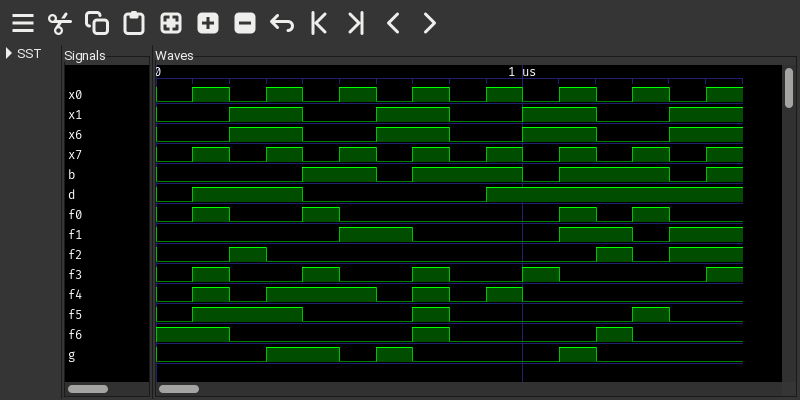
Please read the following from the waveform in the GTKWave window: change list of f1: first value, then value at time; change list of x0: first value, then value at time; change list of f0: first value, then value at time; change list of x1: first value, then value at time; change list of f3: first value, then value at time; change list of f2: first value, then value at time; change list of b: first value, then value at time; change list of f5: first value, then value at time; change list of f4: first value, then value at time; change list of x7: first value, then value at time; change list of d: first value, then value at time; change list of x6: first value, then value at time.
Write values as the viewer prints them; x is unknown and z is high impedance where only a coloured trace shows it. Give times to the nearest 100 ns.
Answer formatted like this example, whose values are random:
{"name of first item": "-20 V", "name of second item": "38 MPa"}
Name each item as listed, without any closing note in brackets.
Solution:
{"change list of f1: first value, then value at time": "0, 1 at 500 ns, 0 at 700 ns, 1 at 1100 ns, 0 at 1300 ns, 1 at 1400 ns", "change list of x0: first value, then value at time": "0, 1 at 100 ns, 0 at 200 ns, 1 at 300 ns, 0 at 400 ns, 1 at 500 ns, 0 at 600 ns, 1 at 700 ns, 0 at 800 ns, 1 at 900 ns, 0 at 1000 ns, 1 at 1100 ns, 0 at 1200 ns, 1 at 1300 ns, 0 at 1400 ns, 1 at 1500 ns", "change list of f0: first value, then value at time": "0, 1 at 100 ns, 0 at 200 ns, 1 at 400 ns, 0 at 500 ns, 1 at 1100 ns, 0 at 1200 ns, 1 at 1300 ns, 0 at 1400 ns", "change list of x1: first value, then value at time": "0, 1 at 200 ns, 0 at 400 ns, 1 at 600 ns, 0 at 800 ns, 1 at 1000 ns, 0 at 1200 ns, 1 at 1400 ns", "change list of f3: first value, then value at time": "0, 1 at 100 ns, 0 at 200 ns, 1 at 400 ns, 0 at 500 ns, 1 at 700 ns, 0 at 800 ns, 1 at 1000 ns, 0 at 1100 ns, 1 at 1500 ns", "change list of f2: first value, then value at time": "0, 1 at 200 ns, 0 at 300 ns, 1 at 1200 ns, 0 at 1300 ns, 1 at 1400 ns", "change list of b: first value, then value at time": "0, 1 at 400 ns, 0 at 600 ns, 1 at 700 ns, 0 at 1000 ns, 1 at 1100 ns, 0 at 1400 ns, 1 at 1500 ns", "change list of f5: first value, then value at time": "0, 1 at 100 ns, 0 at 400 ns, 1 at 700 ns, 0 at 800 ns, 1 at 1300 ns, 0 at 1400 ns", "change list of f4: first value, then value at time": "0, 1 at 100 ns, 0 at 200 ns, 1 at 300 ns, 0 at 600 ns, 1 at 700 ns, 0 at 800 ns, 1 at 900 ns, 0 at 1000 ns", "change list of x7: first value, then value at time": "0, 1 at 100 ns, 0 at 200 ns, 1 at 300 ns, 0 at 400 ns, 1 at 500 ns, 0 at 600 ns, 1 at 700 ns, 0 at 800 ns, 1 at 900 ns, 0 at 1000 ns, 1 at 1100 ns, 0 at 1200 ns, 1 at 1300 ns, 0 at 1400 ns, 1 at 1500 ns", "change list of d: first value, then value at time": "0, 1 at 100 ns, 0 at 400 ns, 1 at 900 ns", "change list of x6: first value, then value at time": "0, 1 at 200 ns, 0 at 400 ns, 1 at 600 ns, 0 at 800 ns, 1 at 1000 ns, 0 at 1200 ns, 1 at 1400 ns"}
